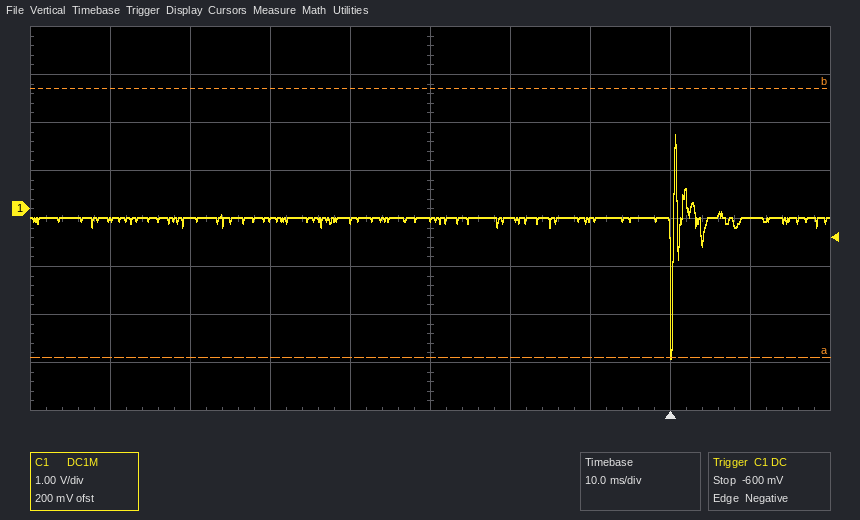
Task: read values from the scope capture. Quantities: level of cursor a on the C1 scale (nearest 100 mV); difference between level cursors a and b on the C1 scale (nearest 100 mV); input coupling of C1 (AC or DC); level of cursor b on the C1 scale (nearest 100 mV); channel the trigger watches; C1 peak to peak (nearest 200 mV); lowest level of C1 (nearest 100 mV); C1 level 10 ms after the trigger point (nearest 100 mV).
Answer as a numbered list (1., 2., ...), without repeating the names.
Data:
1. -3.1 V
2. 5.6 V
3. DC
4. 2.5 V
5. C1
6. 4.6 V
7. -3.1 V
8. -200 mV
